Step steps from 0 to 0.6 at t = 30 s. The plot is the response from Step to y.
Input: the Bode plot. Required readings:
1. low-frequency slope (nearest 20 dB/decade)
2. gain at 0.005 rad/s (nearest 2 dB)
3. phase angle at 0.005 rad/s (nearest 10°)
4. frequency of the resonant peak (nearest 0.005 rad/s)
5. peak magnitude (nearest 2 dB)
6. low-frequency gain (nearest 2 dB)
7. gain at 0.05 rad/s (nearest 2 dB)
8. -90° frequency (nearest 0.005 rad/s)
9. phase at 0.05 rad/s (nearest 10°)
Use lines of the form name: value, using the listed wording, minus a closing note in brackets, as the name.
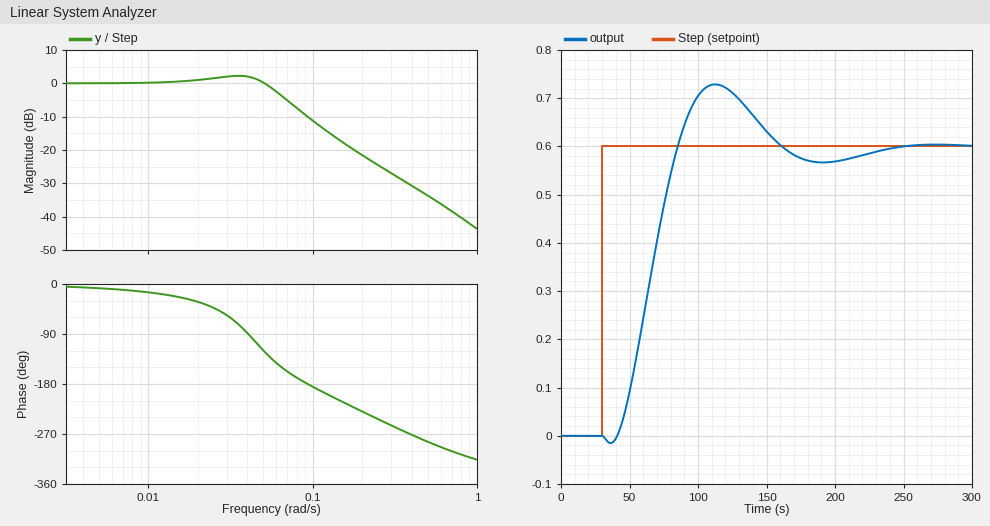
low-frequency slope: 0 dB/decade
gain at 0.005 rad/s: 0 dB
phase angle at 0.005 rad/s: -10°
frequency of the resonant peak: 0.035 rad/s
peak magnitude: 2 dB
low-frequency gain: 0 dB
gain at 0.05 rad/s: 0 dB
-90° frequency: 0.040 rad/s
phase at 0.05 rad/s: -120°
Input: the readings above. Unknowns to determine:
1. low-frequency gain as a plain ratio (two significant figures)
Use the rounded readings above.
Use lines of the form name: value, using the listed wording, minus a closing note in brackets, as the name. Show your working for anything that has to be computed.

low-frequency gain as a plain ratio: 10^(0 / 20) = 1.0
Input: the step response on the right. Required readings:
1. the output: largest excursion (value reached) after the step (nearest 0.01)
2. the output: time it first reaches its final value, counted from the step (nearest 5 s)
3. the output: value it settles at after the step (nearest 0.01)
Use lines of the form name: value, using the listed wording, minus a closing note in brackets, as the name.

the output: largest excursion (value reached) after the step: 0.73
the output: time it first reaches its final value, counted from the step: 55 s
the output: value it settles at after the step: 0.60
